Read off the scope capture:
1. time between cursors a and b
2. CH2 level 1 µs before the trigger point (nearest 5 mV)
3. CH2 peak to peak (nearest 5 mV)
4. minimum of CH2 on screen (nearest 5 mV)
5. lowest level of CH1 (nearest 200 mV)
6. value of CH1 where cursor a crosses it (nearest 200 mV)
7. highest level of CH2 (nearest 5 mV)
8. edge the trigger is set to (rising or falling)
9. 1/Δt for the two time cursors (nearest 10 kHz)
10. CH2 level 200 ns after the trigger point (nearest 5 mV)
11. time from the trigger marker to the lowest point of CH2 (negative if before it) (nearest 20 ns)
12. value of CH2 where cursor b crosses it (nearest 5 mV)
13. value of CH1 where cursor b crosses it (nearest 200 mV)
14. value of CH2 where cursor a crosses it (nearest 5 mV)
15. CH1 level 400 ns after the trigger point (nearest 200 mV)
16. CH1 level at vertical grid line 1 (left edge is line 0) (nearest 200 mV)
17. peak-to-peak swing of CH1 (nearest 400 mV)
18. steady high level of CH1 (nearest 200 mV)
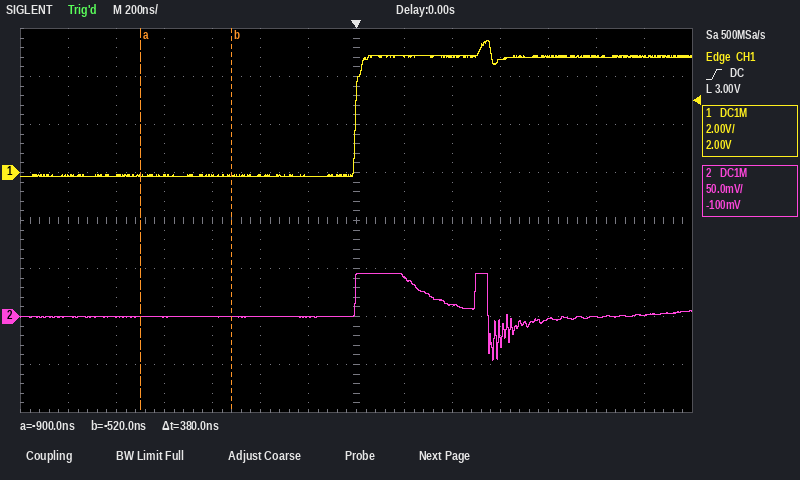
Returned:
380 ns
0 mV
90 mV
-45 mV
-200 mV
-200 mV
45 mV
rising
2.63 MHz
40 mV
+580 ns
0 mV
-200 mV
0 mV
4.8 V
-200 mV
5.6 V
4.8 V
